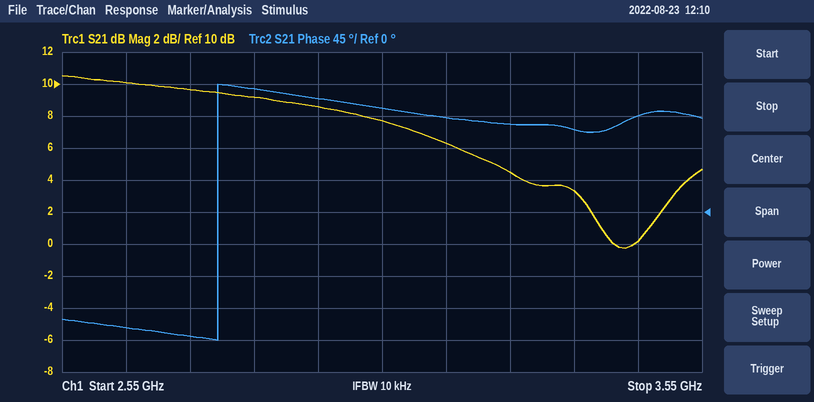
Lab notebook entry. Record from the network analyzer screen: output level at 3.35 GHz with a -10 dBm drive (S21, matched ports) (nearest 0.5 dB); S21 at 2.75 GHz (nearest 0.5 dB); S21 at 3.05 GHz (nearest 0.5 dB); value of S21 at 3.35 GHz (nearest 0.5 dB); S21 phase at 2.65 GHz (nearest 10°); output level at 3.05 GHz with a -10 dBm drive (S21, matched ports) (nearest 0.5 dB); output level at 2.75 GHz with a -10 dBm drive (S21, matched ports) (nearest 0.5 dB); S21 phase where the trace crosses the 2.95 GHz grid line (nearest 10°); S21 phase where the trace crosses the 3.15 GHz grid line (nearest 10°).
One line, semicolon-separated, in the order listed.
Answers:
-6.5 dBm; 9.5 dB; 7.5 dB; 3.5 dB; -160°; -2.5 dBm; -0.5 dBm; 160°; 130°
